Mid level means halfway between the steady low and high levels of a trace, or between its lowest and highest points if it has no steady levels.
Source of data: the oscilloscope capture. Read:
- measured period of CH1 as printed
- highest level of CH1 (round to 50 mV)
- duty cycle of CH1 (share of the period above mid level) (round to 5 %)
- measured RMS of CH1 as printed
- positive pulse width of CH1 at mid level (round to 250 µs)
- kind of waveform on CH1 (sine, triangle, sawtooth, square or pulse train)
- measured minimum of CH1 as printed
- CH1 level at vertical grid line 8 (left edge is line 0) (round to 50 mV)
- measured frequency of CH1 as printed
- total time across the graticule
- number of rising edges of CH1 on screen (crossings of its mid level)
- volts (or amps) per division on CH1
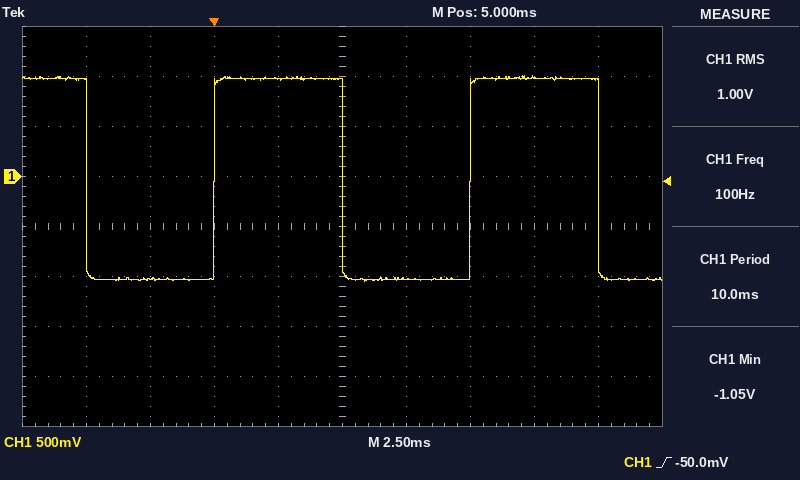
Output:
10.0 ms
1.00 V
50 %
1.00 V
5.00 ms
square
-1.05 V
1.00 V
100 Hz
25 ms
2
500 mV
